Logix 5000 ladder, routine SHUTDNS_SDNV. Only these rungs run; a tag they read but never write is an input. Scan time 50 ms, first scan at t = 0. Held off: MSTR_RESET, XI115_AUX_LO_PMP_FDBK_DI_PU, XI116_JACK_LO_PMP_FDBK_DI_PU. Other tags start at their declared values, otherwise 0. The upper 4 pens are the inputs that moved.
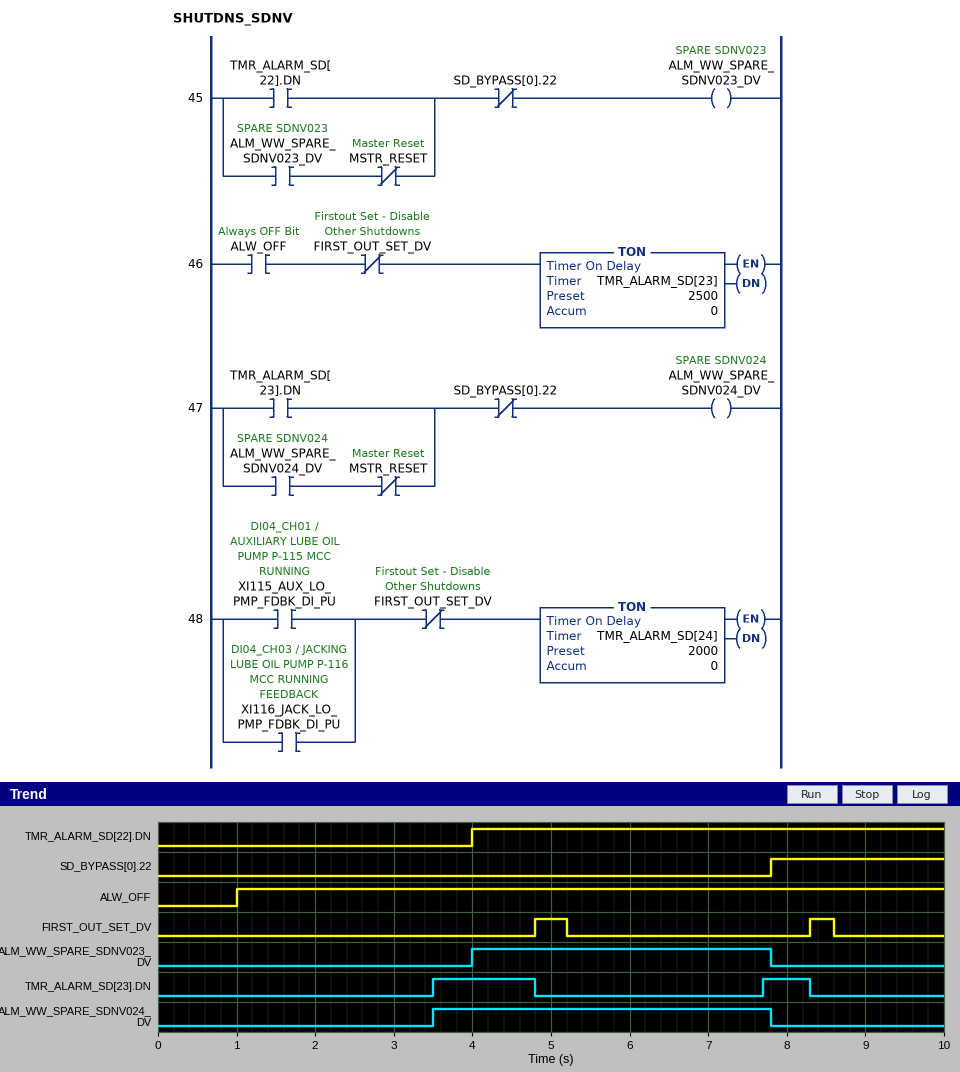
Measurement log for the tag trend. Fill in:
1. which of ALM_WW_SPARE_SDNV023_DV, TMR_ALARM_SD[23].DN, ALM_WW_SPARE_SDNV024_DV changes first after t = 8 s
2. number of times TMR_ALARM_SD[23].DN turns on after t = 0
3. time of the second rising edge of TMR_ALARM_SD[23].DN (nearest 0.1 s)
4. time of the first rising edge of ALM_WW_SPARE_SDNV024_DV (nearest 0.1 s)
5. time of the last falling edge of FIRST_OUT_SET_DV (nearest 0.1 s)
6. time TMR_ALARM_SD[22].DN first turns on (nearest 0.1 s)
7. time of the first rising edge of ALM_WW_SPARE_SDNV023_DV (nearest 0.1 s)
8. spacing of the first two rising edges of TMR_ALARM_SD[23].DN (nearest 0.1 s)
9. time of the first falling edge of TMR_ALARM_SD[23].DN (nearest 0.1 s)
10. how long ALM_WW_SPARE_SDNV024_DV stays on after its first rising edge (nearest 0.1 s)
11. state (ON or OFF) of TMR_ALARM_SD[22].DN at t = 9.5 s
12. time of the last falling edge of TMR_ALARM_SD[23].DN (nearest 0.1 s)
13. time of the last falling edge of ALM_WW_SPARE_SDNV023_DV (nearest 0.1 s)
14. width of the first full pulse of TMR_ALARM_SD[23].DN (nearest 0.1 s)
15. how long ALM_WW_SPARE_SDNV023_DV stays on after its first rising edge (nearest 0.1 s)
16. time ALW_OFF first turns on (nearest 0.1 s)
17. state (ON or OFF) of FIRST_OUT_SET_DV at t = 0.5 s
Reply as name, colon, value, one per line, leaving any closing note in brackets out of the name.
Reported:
which of ALM_WW_SPARE_SDNV023_DV, TMR_ALARM_SD[23].DN, ALM_WW_SPARE_SDNV024_DV changes first after t = 8 s: TMR_ALARM_SD[23].DN
number of times TMR_ALARM_SD[23].DN turns on after t = 0: 2
time of the second rising edge of TMR_ALARM_SD[23].DN: 7.7 s
time of the first rising edge of ALM_WW_SPARE_SDNV024_DV: 3.5 s
time of the last falling edge of FIRST_OUT_SET_DV: 8.6 s
time TMR_ALARM_SD[22].DN first turns on: 4.0 s
time of the first rising edge of ALM_WW_SPARE_SDNV023_DV: 4.0 s
spacing of the first two rising edges of TMR_ALARM_SD[23].DN: 4.2 s
time of the first falling edge of TMR_ALARM_SD[23].DN: 4.8 s
how long ALM_WW_SPARE_SDNV024_DV stays on after its first rising edge: 4.3 s
state (ON or OFF) of TMR_ALARM_SD[22].DN at t = 9.5 s: ON
time of the last falling edge of TMR_ALARM_SD[23].DN: 8.3 s
time of the last falling edge of ALM_WW_SPARE_SDNV023_DV: 7.8 s
width of the first full pulse of TMR_ALARM_SD[23].DN: 1.3 s
how long ALM_WW_SPARE_SDNV023_DV stays on after its first rising edge: 3.8 s
time ALW_OFF first turns on: 1.0 s
state (ON or OFF) of FIRST_OUT_SET_DV at t = 0.5 s: OFF
